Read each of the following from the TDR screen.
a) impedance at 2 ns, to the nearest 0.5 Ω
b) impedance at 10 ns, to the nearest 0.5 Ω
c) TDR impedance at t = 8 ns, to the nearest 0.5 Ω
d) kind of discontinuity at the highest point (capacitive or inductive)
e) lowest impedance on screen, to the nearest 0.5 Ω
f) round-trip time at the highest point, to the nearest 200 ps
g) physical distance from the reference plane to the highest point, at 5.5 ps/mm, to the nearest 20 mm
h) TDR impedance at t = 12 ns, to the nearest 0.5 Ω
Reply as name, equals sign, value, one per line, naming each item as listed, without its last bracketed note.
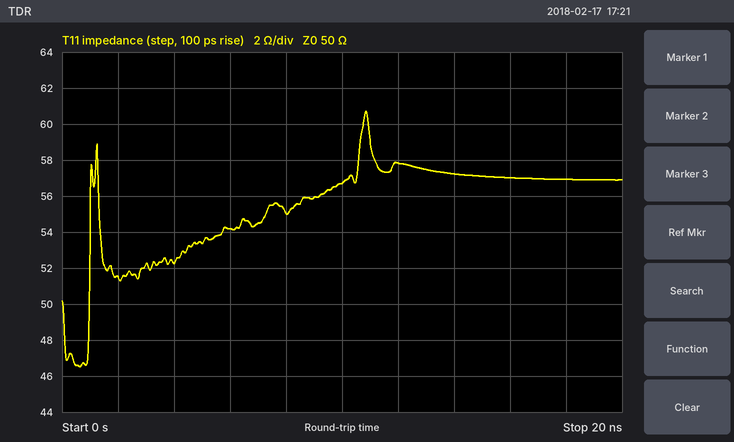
impedance at 2 ns, to the nearest 0.5 Ω = 51.5 Ω
impedance at 10 ns, to the nearest 0.5 Ω = 56.5 Ω
TDR impedance at t = 8 ns, to the nearest 0.5 Ω = 55.0 Ω
kind of discontinuity at the highest point = inductive
lowest impedance on screen, to the nearest 0.5 Ω = 46.5 Ω
round-trip time at the highest point, to the nearest 200 ps = 10.8 ns
physical distance from the reference plane to the highest point, at 5.5 ps/mm, to the nearest 20 mm = 980 mm
TDR impedance at t = 12 ns, to the nearest 0.5 Ω = 58.0 Ω
